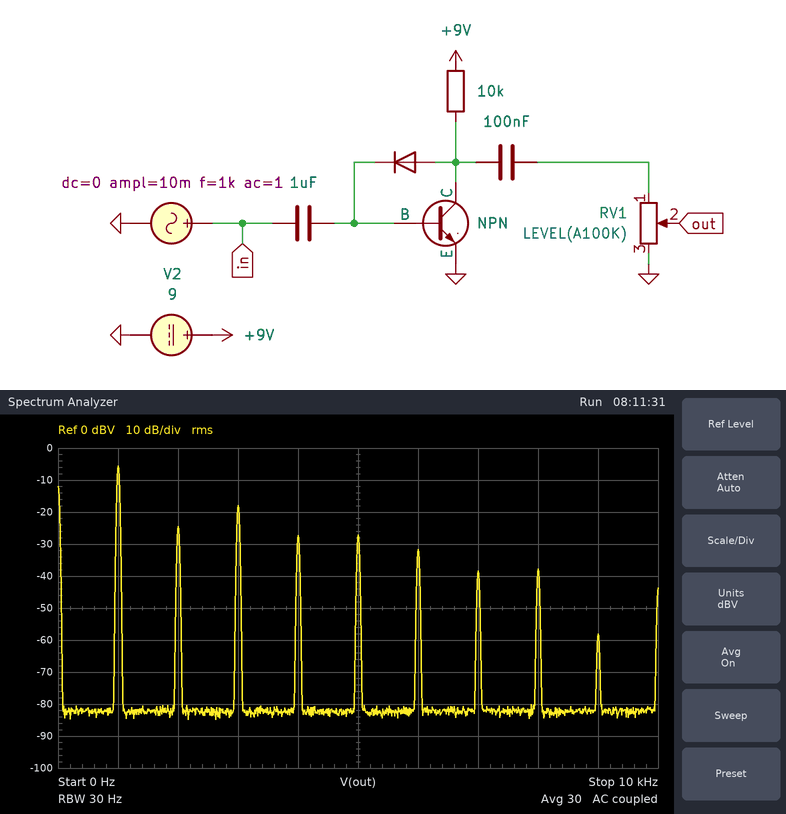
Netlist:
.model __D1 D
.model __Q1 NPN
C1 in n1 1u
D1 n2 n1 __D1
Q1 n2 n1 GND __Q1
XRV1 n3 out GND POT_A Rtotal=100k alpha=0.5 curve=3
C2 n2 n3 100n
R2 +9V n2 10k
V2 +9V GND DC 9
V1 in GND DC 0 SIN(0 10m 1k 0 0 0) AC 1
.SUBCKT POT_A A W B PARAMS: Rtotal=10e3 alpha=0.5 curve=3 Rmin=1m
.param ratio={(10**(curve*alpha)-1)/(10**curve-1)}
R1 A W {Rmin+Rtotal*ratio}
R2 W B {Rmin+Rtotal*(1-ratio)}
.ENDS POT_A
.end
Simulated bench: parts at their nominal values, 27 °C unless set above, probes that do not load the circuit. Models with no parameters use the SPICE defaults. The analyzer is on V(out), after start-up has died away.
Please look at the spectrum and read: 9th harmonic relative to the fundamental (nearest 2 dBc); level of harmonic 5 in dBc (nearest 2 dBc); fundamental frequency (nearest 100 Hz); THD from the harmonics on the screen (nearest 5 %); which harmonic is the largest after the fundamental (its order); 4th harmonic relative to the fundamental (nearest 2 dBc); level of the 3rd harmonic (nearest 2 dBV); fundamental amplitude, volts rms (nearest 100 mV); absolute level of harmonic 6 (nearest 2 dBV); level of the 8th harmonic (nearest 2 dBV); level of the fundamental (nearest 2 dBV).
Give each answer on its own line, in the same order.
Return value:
-52 dBc
-22 dBc
1.0 kHz
30 %
3
-22 dBc
-18 dBV
500 mV
-32 dBV
-38 dBV
-6 dBV
